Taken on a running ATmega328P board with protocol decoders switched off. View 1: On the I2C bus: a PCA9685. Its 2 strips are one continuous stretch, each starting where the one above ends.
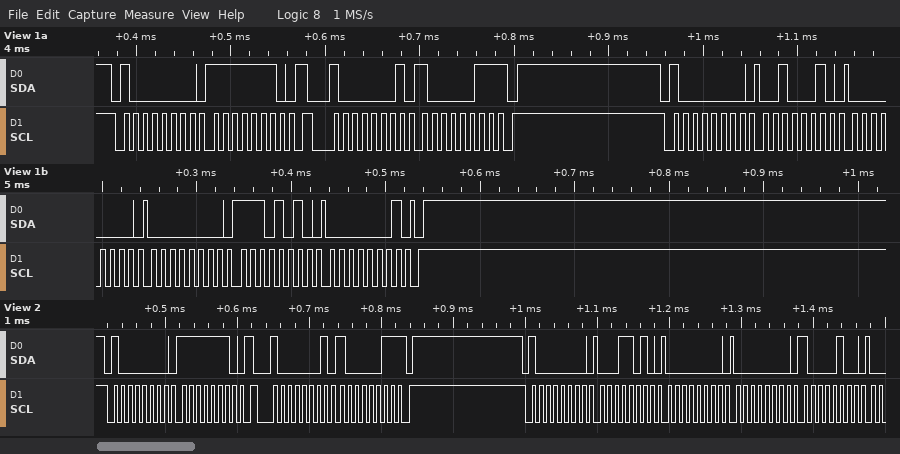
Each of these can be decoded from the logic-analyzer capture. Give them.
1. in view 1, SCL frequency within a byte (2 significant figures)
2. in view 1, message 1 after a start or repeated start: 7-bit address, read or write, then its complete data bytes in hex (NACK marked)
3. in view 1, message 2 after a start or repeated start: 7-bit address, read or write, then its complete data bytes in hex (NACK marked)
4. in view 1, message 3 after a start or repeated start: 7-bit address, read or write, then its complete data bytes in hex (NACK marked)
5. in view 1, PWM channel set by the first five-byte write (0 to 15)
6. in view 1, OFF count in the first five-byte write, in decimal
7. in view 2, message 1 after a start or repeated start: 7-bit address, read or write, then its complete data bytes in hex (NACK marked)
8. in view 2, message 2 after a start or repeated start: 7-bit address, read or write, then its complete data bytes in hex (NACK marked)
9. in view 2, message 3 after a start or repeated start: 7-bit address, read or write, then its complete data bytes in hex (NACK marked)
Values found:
100 kHz
0x40 write: FE
0x40 read: 83 NACK
0x40 write: 22 00 00 EA 01
7
490
0x40 write: FE
0x40 read: 83 NACK
0x40 write: 1A 00 00 84
